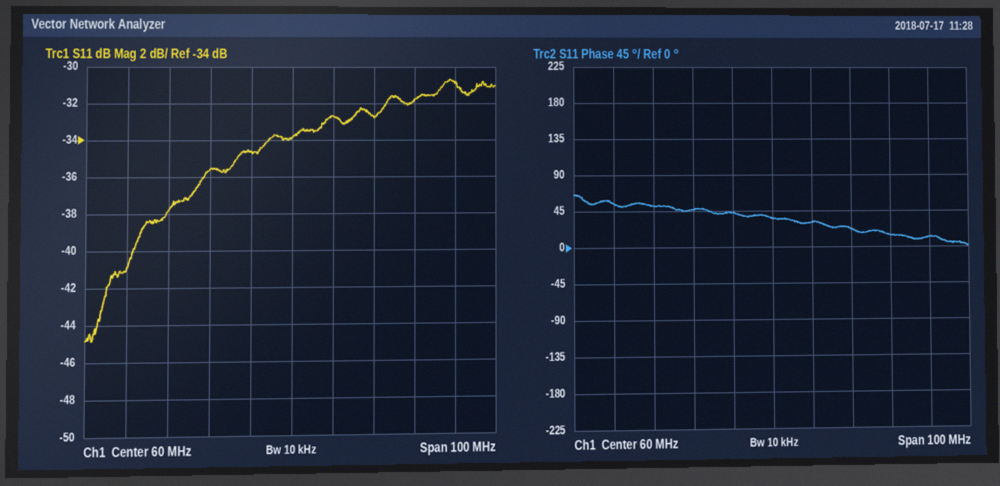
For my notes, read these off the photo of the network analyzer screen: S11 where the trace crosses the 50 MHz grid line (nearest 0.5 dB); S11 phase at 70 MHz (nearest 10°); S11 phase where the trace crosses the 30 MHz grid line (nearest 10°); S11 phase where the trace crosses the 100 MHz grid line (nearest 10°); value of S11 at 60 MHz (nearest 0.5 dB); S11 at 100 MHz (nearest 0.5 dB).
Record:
-34.5 dB
30°
50°
10°
-34.0 dB
-31.0 dB
